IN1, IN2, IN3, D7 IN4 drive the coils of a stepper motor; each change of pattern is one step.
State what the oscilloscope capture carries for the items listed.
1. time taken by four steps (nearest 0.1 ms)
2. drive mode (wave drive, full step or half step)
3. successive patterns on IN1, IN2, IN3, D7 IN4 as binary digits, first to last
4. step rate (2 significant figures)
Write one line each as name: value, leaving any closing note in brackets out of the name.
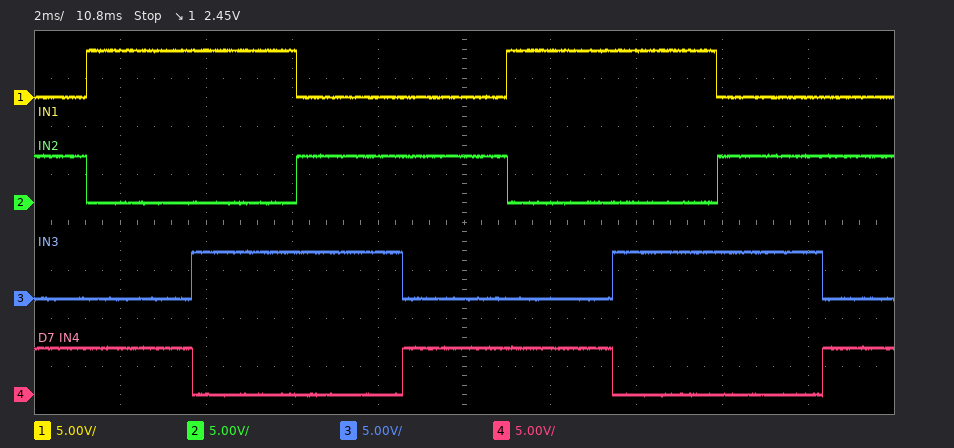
time taken by four steps: 9.8 ms
drive mode: full step
successive patterns on IN1, IN2, IN3, D7 IN4 as binary digits, first to last: 0101 1001 1010 0110 0101 1001 1010 0110 0101
step rate: 410 steps/s
